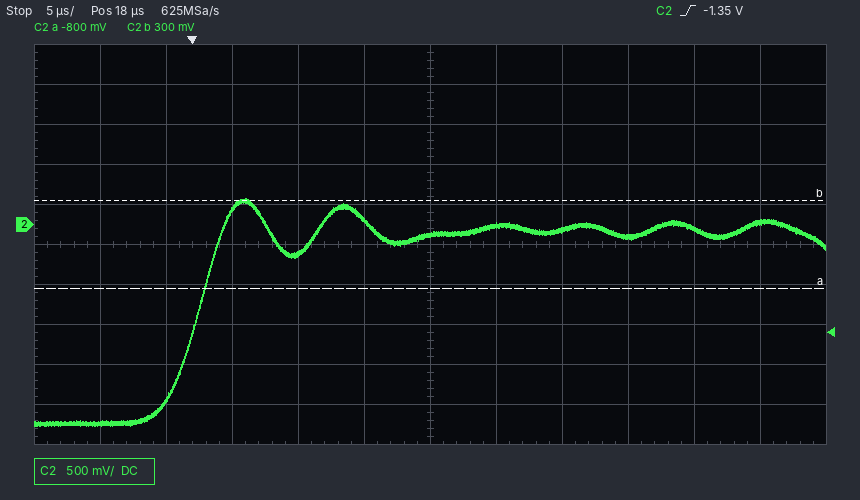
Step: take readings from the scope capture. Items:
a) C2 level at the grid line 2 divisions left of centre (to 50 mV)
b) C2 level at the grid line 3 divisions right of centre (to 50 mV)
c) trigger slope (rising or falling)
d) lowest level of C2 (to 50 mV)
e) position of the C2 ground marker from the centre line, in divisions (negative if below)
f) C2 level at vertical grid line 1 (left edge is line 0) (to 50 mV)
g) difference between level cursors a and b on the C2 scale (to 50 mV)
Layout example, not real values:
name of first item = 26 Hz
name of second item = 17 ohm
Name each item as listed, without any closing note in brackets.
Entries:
C2 level at the grid line 2 divisions left of centre = -350 mV
C2 level at the grid line 3 divisions right of centre = -150 mV
trigger slope = rising
lowest level of C2 = -2.50 V
position of the C2 ground marker from the centre line, in divisions = +0.5 div
C2 level at vertical grid line 1 (left edge is line 0) = -2.50 V
difference between level cursors a and b on the C2 scale = 1.10 V
